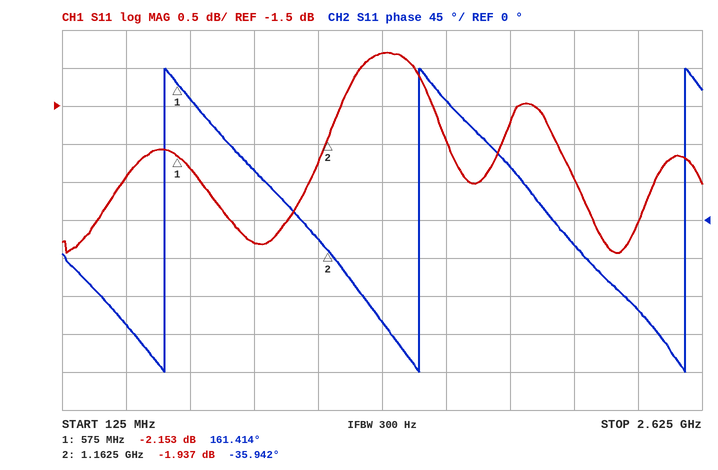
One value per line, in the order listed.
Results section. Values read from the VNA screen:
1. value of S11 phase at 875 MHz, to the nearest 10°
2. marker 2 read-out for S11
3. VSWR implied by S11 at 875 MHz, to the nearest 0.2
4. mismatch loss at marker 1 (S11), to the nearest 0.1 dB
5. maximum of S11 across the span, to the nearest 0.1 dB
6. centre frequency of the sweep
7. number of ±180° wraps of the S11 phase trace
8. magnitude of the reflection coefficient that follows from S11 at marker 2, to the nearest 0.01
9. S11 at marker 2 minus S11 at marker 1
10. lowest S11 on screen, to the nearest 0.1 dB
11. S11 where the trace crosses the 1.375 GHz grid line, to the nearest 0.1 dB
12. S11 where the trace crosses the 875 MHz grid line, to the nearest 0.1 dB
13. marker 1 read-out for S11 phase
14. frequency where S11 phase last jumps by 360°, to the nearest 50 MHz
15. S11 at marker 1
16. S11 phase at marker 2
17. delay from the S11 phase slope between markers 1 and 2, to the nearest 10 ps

60°
-1.937 dB
5.4
4.1 dB
-0.8 dB
1.375 GHz
3
0.80
0.216 dB
-3.4 dB
-0.8 dB
-3.3 dB
161.414°
2.55 GHz
-2.153 dB
-35.942°
930 ps
